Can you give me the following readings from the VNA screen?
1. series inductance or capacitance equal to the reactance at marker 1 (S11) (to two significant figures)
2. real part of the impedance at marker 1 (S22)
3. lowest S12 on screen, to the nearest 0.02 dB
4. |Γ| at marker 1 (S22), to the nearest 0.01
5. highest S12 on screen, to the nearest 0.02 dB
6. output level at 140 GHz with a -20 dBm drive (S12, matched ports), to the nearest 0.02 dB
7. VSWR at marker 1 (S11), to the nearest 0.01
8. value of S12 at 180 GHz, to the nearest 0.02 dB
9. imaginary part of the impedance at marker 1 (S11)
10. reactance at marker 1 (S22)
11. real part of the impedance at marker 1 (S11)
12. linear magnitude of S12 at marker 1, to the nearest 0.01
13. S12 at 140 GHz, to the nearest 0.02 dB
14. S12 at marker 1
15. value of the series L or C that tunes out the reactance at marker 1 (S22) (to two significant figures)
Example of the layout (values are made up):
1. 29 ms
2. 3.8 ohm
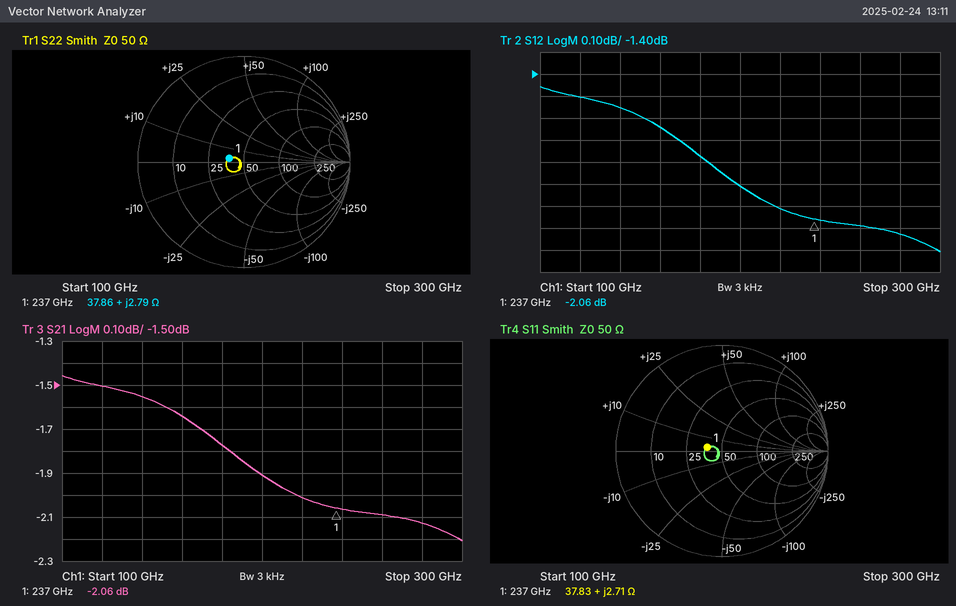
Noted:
1. 1.8 pH
2. 37.86 Ω
3. -2.20 dB
4. 0.14
5. -1.46 dB
6. -21.56 dBm
7. 1.33
8. -1.78 dB
9. +2.71 Ω
10. +2.79 Ω
11. 37.83 Ω
12. 0.79
13. -1.56 dB
14. -2.06 dB
15. 240 fF
